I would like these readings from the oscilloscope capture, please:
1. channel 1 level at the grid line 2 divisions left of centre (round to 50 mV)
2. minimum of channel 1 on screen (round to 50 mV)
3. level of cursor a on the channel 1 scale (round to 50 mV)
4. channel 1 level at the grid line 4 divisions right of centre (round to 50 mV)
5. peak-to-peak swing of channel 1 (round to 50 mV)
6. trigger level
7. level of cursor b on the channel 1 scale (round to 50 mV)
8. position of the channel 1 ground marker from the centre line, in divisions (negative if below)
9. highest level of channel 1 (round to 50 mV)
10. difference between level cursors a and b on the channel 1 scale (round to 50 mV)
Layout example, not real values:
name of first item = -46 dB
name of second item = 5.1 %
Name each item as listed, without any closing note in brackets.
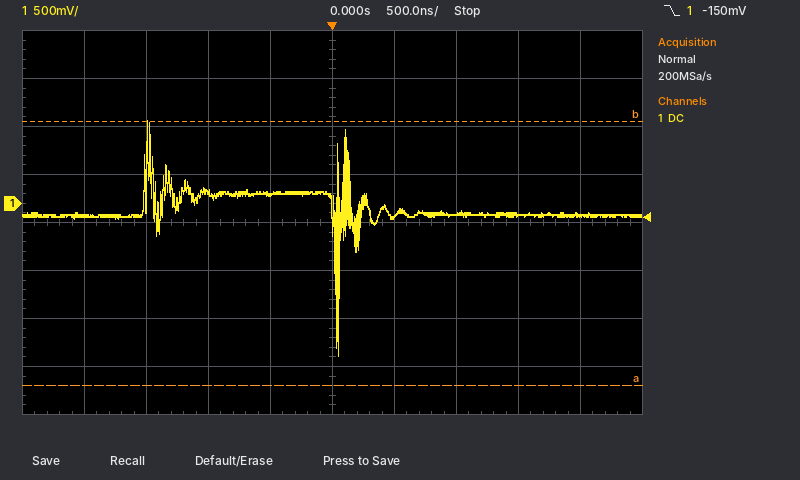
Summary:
channel 1 level at the grid line 2 divisions left of centre = 100 mV
minimum of channel 1 on screen = -1.60 V
level of cursor a on the channel 1 scale = -1.90 V
channel 1 level at the grid line 4 divisions right of centre = -100 mV
peak-to-peak swing of channel 1 = 2.45 V
trigger level = -150 mV
level of cursor b on the channel 1 scale = 850 mV
position of the channel 1 ground marker from the centre line, in divisions = +0.4 div
highest level of channel 1 = 850 mV
difference between level cursors a and b on the channel 1 scale = 2.75 V
